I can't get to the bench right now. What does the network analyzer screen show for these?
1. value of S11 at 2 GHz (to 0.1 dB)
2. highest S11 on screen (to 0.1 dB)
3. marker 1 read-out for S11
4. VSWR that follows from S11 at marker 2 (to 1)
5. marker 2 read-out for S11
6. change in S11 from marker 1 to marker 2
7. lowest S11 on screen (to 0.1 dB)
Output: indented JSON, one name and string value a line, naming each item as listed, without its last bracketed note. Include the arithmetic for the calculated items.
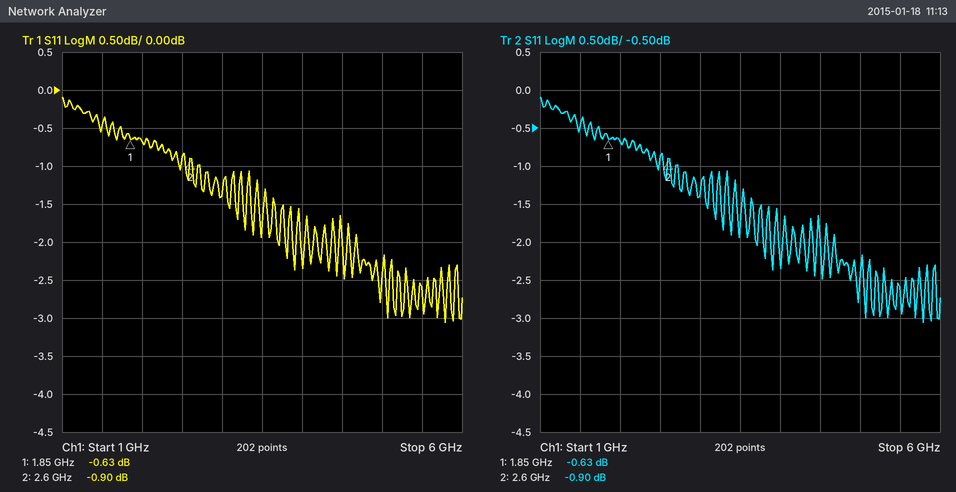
{
  "value of S11 at 2 GHz": "-0.7 dB",
  "highest S11 on screen": "-0.1 dB",
  "marker 1 read-out for S11": "-0.63 dB",
  "VSWR that follows from S11 at marker 2": "(1 + 0.9016)/(1 − 0.9016) ≈ 19",
  "marker 2 read-out for S11": "-0.90 dB",
  "change in S11 from marker 1 to marker 2": "-0.9 − (-0.63) = -0.27 dB",
  "lowest S11 on screen": "-3.1 dB"
}
